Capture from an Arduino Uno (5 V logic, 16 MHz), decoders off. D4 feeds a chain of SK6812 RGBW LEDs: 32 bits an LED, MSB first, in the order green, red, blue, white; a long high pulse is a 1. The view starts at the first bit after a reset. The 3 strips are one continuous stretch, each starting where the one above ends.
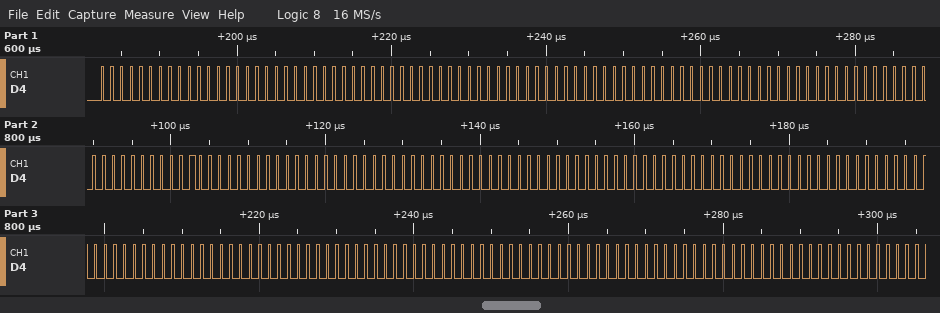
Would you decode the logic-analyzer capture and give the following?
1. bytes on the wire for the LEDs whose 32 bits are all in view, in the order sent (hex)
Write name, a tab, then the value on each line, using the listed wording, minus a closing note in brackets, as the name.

bytes on the wire for the LEDs whose 32 bits are all in view, in the order sent	00 00 00 00 00 00 00 00 00 00 00 00 80 00 00 00 00 00 00 00 00 00 00 00 00 00 00 00 00 00 00 00
